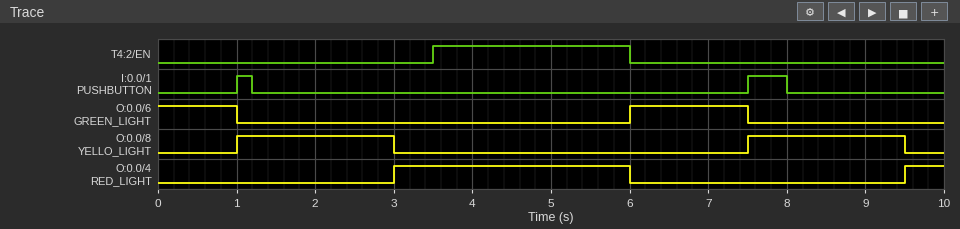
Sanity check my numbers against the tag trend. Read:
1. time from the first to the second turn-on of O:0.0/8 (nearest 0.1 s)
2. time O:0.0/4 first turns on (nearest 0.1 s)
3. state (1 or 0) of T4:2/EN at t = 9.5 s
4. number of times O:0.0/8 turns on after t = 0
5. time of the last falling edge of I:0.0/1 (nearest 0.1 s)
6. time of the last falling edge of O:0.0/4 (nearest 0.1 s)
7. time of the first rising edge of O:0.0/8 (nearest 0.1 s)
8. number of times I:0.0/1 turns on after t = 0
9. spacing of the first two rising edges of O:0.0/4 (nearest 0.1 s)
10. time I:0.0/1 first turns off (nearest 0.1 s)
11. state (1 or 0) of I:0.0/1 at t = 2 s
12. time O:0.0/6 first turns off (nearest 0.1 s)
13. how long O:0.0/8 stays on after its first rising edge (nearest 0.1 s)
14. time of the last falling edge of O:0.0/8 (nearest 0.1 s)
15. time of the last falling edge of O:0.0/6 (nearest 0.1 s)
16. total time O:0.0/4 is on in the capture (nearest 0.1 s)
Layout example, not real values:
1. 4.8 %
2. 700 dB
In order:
1. 6.5 s
2. 3.0 s
3. 0
4. 2
5. 8.0 s
6. 6.0 s
7. 1.0 s
8. 2
9. 6.5 s
10. 1.2 s
11. 0
12. 1.0 s
13. 2.0 s
14. 9.5 s
15. 7.5 s
16. 3.5 s
